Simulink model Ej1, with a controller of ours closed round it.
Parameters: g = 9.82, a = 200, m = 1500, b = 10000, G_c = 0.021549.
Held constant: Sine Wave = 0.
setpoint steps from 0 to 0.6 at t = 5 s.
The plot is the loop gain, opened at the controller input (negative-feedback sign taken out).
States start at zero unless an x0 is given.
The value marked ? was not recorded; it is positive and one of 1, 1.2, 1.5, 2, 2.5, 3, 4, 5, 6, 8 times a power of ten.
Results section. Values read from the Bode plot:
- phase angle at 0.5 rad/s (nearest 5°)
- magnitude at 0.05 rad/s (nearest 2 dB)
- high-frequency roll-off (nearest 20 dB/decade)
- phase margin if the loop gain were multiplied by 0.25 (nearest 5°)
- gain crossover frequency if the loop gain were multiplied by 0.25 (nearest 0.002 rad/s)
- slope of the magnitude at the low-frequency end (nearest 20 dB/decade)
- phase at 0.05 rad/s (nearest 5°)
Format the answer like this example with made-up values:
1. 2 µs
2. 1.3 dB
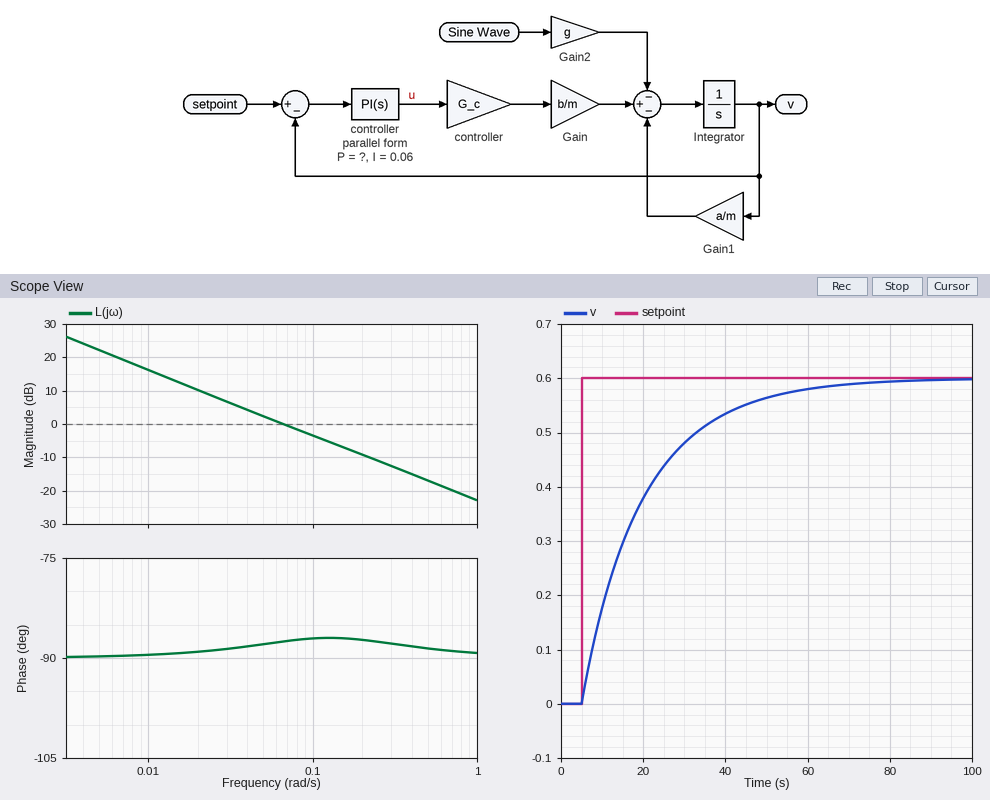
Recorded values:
1. -90°
2. 2 dB
3. -20 dB/decade
4. 90°
5. 0.016 rad/s
6. -20 dB/decade
7. -90°
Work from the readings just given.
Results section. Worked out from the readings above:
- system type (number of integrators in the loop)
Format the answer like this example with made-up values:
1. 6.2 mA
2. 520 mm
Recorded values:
1. 1
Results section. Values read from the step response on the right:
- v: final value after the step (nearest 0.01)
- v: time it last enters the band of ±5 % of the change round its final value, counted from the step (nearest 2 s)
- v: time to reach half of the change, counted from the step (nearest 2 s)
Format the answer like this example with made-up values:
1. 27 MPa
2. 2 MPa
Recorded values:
1. 0.60
2. 48 s
3. 10 s
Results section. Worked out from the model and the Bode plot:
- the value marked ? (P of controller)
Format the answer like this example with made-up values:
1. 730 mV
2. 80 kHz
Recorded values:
1. 0.5
